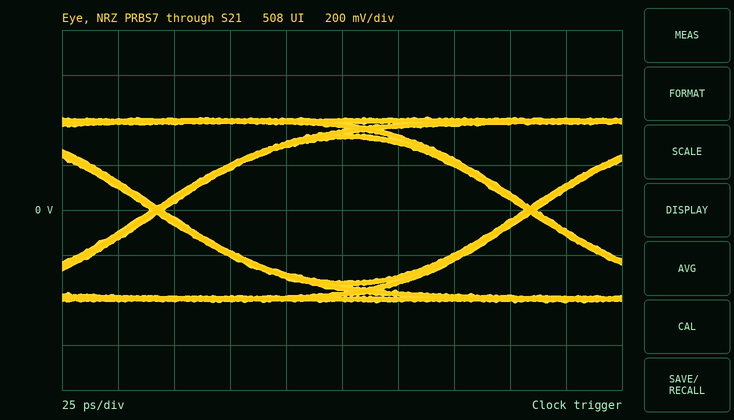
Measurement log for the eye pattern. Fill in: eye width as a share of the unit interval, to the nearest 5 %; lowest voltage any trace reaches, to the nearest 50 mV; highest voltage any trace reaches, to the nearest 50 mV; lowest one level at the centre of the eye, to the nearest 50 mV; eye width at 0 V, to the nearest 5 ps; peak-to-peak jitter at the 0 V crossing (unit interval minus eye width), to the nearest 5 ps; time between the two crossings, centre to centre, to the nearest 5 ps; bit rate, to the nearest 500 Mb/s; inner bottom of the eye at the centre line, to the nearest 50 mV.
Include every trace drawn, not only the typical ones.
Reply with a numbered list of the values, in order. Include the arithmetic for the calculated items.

1. 160 ps / 165 ps ≈ 97.0 %, so 95 % to the nearest 5 %
2. -400 mV
3. 400 mV
4. 300 mV
5. 160 ps
6. 5 ps
7. 165 ps
8. 6.0 Gb/s
9. -300 mV
